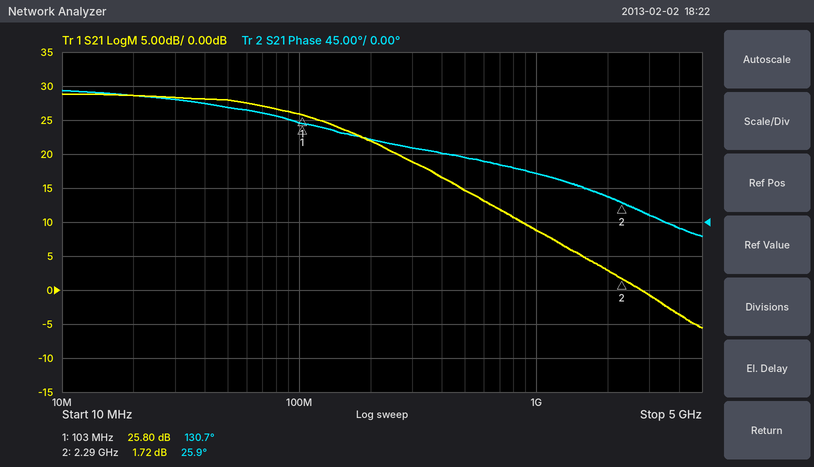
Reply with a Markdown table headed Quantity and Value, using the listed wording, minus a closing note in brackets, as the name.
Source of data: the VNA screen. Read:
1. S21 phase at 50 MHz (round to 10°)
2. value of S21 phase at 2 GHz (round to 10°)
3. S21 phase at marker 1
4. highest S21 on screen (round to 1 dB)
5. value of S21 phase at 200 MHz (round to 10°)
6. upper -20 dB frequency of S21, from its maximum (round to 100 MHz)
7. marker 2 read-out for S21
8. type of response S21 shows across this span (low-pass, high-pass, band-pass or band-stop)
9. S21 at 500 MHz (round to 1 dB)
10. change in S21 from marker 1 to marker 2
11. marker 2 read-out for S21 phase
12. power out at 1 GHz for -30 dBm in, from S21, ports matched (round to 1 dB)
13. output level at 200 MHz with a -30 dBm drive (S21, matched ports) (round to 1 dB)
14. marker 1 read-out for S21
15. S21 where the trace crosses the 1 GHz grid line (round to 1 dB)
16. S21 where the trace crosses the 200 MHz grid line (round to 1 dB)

| Quantity | Value |
|---|---|
| S21 phase at 50 MHz | 150° |
| value of S21 phase at 2 GHz | 30° |
| S21 phase at marker 1 | 130.7° |
| highest S21 on screen | 29 dB |
| value of S21 phase at 200 MHz | 110° |
| upper -20 dB frequency of S21, from its maximum | 1.0 GHz |
| marker 2 read-out for S21 | 1.72 dB |
| type of response S21 shows across this span | low-pass |
| S21 at 500 MHz | 15 dB |
| change in S21 from marker 1 to marker 2 | -24.08 dB |
| marker 2 read-out for S21 phase | 25.9° |
| power out at 1 GHz for -30 dBm in, from S21, ports matched | -21 dBm |
| output level at 200 MHz with a -30 dBm drive (S21, matched ports) | -8 dBm |
| marker 1 read-out for S21 | 25.80 dB |
| S21 where the trace crosses the 1 GHz grid line | 9 dB |
| S21 where the trace crosses the 200 MHz grid line | 22 dB |
